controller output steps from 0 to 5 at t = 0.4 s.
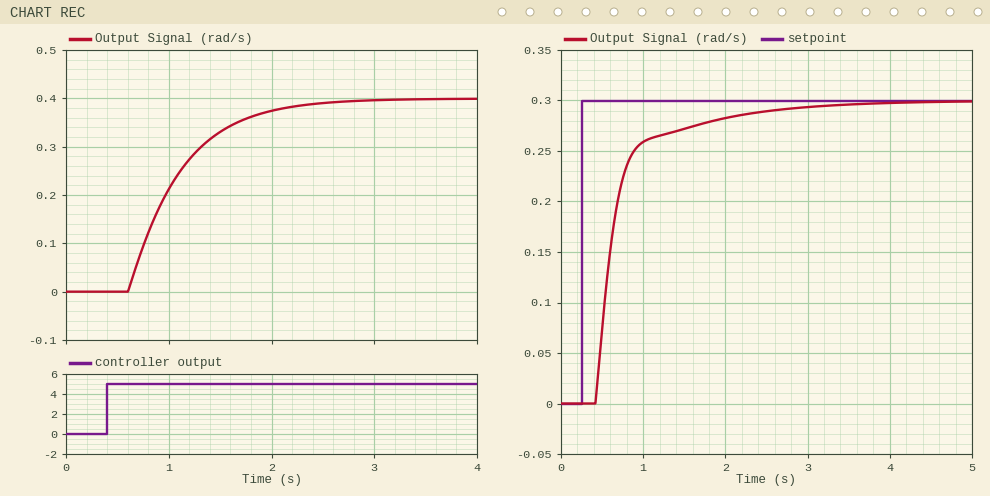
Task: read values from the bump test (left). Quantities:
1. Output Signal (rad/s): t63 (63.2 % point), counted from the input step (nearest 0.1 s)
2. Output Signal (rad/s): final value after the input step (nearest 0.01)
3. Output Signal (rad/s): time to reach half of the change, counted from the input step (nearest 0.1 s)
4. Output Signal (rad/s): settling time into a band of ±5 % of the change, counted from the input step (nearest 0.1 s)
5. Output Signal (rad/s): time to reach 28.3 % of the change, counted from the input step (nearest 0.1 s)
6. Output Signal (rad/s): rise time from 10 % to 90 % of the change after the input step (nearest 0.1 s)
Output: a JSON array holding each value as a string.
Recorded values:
["0.7 s", "0.40", "0.6 s", "1.7 s", "0.4 s", "1.1 s"]
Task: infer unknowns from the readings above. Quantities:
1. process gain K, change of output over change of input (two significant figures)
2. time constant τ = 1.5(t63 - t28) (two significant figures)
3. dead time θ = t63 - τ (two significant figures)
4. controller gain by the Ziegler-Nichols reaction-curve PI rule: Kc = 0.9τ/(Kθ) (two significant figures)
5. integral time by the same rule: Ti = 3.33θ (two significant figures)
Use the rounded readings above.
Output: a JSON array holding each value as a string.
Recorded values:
["0.080", "0.45 s", "0.25 s", "20", "0.83 s"]
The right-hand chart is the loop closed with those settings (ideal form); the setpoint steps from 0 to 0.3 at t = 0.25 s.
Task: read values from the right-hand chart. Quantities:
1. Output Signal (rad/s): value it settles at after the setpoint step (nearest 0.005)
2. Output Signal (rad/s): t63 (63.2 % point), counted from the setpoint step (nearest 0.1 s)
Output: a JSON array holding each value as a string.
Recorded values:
["0.300", "0.4 s"]
